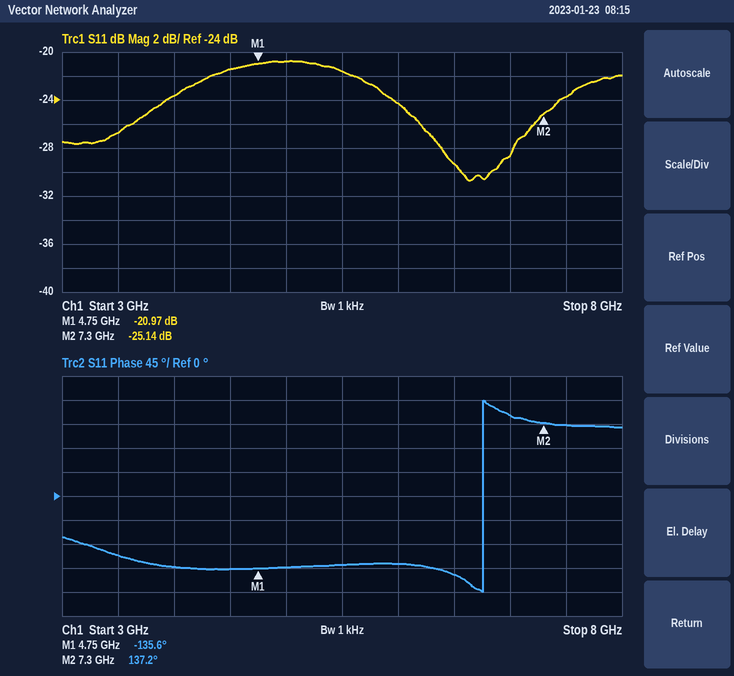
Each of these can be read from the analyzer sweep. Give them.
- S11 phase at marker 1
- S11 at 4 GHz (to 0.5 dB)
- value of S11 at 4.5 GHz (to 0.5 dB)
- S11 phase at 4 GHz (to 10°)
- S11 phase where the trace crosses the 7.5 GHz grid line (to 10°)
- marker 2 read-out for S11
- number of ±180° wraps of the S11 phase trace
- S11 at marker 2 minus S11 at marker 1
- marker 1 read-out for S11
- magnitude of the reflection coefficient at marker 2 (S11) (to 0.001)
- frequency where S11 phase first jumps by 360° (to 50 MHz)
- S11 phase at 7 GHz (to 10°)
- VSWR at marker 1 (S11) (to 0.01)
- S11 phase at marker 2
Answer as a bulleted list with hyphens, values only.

- -135.6°
- -23.5 dB
- -21.5 dB
- -130°
- 130°
- -25.14 dB
- 1
- -4.17 dB
- -20.97 dB
- 0.055
- 6.75 GHz
- 150°
- 1.20
- 137.2°
